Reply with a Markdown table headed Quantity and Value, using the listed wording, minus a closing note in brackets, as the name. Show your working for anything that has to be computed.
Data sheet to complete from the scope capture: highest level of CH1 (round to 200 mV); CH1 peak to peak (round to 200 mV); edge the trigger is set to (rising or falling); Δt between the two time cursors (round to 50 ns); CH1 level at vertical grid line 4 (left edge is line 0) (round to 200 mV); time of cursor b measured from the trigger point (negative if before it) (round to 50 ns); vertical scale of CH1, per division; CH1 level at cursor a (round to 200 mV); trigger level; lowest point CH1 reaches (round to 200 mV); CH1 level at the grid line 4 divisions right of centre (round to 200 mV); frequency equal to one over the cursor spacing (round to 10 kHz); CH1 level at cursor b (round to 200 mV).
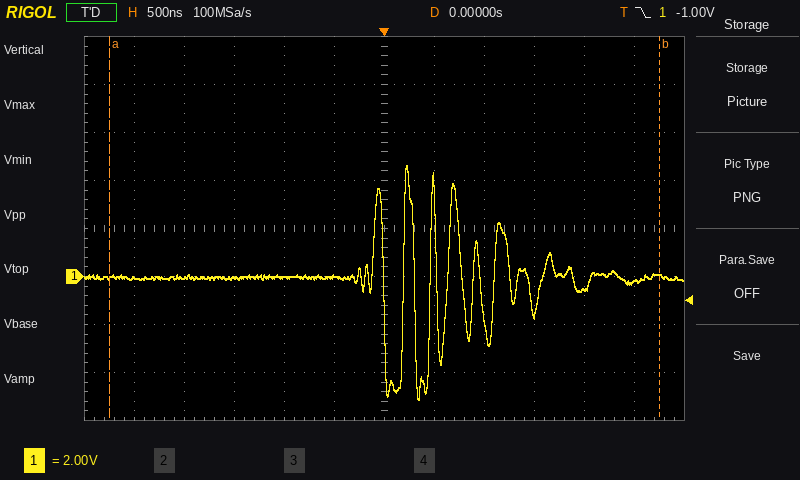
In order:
| Quantity | Value |
|---|---|
| highest level of CH1 | 4.6 V |
| CH1 peak to peak | 4.6 V − (-5.2 V) = 9.8 V |
| edge the trigger is set to | falling |
| Δt between the two time cursors | 5.50 µs |
| CH1 level at vertical grid line 4 (left edge is line 0) | 0.0 V |
| time of cursor b measured from the trigger point (negative if before it) | +2.75 µs |
| vertical scale of CH1, per division | 2 V |
| CH1 level at cursor a | 0.0 V |
| trigger level | -1.00 V |
| lowest point CH1 reaches | -5.2 V |
| CH1 level at the grid line 4 divisions right of centre | -600 mV |
| frequency equal to one over the cursor spacing | 1 / 5.50 µs ≈ 180 kHz |
| CH1 level at cursor b | 0.0 V |
